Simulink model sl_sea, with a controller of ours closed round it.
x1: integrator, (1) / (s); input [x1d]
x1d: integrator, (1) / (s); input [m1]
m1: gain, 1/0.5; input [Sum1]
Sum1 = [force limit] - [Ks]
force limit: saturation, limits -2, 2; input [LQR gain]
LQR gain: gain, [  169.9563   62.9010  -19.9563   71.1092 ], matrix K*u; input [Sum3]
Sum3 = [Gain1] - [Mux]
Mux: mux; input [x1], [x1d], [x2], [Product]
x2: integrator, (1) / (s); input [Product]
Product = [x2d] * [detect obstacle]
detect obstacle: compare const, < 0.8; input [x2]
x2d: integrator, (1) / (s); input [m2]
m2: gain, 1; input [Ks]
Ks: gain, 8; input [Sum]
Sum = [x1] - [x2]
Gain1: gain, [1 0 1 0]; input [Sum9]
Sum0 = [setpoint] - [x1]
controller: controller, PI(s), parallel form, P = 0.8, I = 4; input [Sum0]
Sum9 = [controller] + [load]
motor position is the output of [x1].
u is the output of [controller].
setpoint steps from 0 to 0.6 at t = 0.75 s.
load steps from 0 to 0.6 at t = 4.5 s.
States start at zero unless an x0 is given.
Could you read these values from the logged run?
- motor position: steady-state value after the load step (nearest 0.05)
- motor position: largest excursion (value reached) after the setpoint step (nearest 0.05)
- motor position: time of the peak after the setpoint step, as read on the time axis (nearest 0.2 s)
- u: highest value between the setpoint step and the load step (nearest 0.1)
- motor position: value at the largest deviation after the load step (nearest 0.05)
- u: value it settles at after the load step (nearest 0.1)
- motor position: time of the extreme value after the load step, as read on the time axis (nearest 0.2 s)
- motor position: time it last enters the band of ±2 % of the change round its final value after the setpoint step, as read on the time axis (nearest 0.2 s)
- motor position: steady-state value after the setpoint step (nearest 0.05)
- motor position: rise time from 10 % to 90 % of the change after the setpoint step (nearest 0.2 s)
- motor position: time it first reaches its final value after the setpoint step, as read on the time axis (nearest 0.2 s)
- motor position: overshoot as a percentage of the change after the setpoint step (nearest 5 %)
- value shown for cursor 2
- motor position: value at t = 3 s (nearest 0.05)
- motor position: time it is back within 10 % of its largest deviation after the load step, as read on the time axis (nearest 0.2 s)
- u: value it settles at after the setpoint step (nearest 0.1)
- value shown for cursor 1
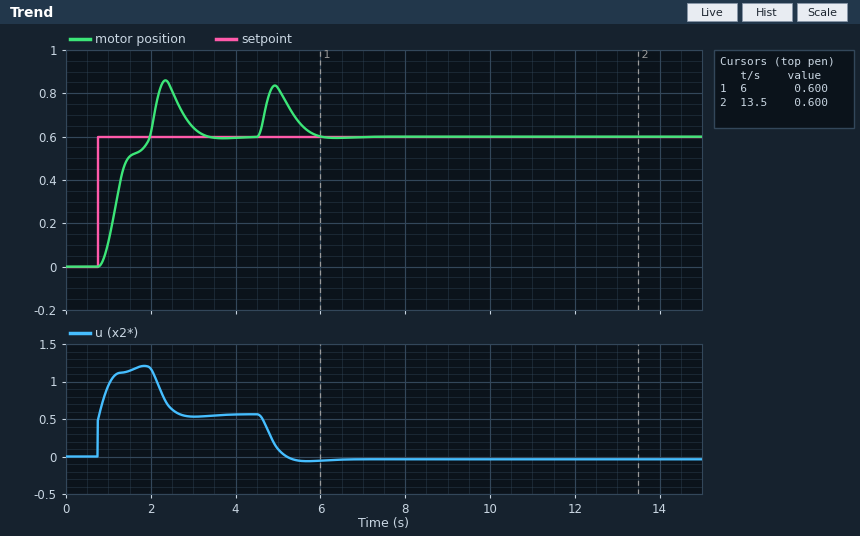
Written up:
0.60
0.85
2.4 s
1.2
0.85
0.0
5.0 s
3.2 s
0.60
0.8 s
2.0 s
45 %
0.600
0.65
5.8 s
0.6
0.600
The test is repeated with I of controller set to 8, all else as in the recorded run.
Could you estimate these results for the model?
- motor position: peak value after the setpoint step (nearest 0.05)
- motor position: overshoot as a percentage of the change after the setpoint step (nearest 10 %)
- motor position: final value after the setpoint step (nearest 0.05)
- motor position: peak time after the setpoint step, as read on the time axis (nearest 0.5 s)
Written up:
0.95
60 %
0.60
2.0 s
